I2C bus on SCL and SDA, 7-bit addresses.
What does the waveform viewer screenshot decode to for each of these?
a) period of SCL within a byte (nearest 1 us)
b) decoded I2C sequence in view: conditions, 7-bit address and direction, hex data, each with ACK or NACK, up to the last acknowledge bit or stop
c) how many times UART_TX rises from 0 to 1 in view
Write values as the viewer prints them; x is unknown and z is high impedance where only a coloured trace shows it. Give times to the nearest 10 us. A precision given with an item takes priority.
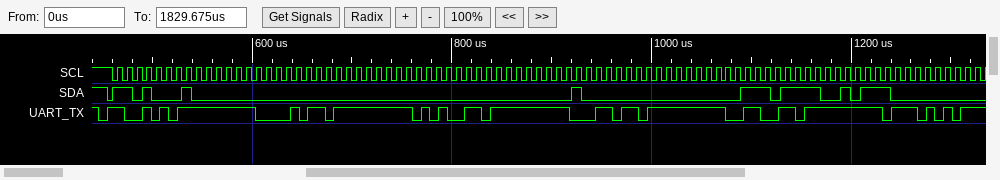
10 us
start, address 68 read ACK, 00 ACK, 00 ACK, 00 ACK, 00 ACK, 40 ACK, 00 ACK, EF ACK, 5C ACK
21
